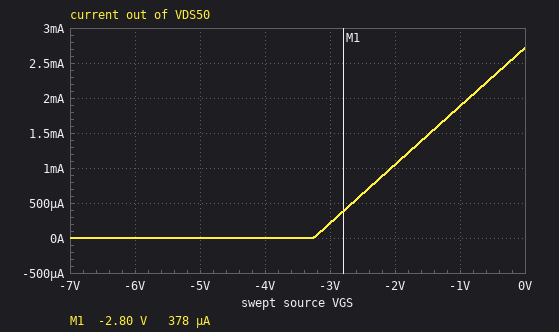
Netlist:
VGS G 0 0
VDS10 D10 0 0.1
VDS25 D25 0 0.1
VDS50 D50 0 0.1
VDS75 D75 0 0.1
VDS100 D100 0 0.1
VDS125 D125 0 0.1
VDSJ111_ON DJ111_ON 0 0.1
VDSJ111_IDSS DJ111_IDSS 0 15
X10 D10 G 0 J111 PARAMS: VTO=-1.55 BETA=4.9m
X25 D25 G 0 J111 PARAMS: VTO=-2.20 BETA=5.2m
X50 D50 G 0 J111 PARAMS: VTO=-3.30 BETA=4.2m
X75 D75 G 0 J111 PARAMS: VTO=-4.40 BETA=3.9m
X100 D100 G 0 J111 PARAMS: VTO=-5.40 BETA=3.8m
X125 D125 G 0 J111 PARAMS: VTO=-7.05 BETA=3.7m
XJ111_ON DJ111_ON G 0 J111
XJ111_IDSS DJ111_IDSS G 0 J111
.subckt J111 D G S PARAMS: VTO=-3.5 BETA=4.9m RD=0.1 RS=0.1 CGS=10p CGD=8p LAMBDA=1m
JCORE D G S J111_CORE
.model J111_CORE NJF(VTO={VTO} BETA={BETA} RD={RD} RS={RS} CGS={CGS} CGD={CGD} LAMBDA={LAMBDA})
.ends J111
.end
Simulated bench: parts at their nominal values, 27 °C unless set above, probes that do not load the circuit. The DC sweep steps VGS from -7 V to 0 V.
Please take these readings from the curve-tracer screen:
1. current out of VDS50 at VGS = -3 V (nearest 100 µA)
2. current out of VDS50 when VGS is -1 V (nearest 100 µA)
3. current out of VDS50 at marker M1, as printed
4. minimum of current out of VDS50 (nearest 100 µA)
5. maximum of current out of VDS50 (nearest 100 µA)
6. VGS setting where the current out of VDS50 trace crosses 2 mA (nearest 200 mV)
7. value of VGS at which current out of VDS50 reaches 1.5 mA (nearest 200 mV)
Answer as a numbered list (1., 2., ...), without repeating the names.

1. 200 µA
2. 1.9 mA
3. 378 µA
4. 0 A
5. 2.7 mA
6. -800 mV
7. -1.4 V
